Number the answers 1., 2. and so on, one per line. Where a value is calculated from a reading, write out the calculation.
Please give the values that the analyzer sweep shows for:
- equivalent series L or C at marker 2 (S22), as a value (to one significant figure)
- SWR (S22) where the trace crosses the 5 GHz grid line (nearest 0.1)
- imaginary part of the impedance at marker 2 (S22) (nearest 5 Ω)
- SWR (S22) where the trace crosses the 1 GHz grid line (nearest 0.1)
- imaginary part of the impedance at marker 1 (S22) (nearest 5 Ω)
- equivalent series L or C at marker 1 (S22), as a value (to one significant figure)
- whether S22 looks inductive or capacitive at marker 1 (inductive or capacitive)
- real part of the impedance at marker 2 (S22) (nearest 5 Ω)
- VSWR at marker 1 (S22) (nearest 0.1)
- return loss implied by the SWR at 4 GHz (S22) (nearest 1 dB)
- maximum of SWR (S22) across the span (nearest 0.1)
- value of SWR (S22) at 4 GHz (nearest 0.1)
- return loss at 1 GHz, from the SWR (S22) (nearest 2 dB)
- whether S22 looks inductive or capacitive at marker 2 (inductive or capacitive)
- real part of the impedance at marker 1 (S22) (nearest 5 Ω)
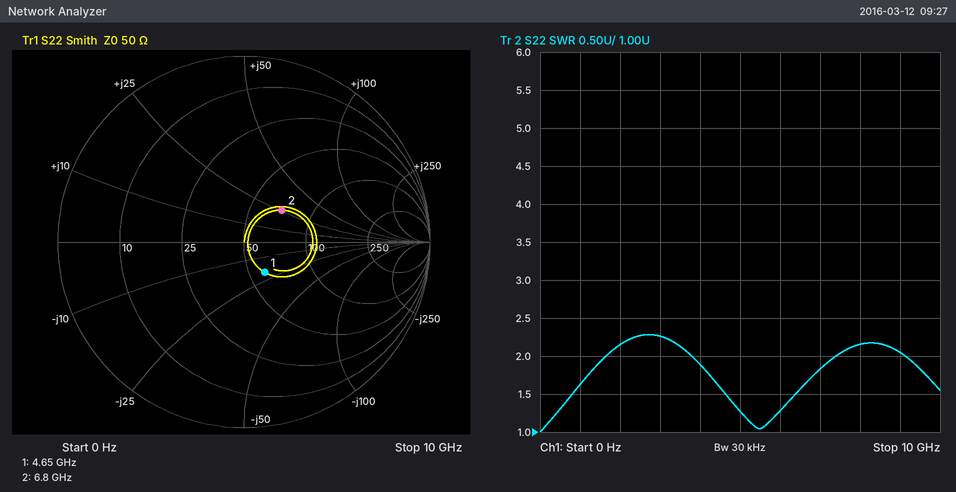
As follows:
1. L = 25 Ω/(2π × 6.8 GHz) ≈ 585 pH, so 600 pH to one significant figure
2. 1.3
3. +25 Ω
4. 1.6
5. -20 Ω
6. C = 1/(2π × 4.65 GHz × 20 Ω) ≈ 2 pF
7. capacitive
8. 70 Ω
9. 1.5
10. −20 log10((1.9 − 1)/(1.9 + 1)) ≈ 10 dB
11. 2.3
12. 1.9
13. −20 log10((1.6 − 1)/(1.6 + 1)) ≈ 12.7 dB, so 12 dB to the nearest 2 dB
14. inductive
15. 60 Ω
